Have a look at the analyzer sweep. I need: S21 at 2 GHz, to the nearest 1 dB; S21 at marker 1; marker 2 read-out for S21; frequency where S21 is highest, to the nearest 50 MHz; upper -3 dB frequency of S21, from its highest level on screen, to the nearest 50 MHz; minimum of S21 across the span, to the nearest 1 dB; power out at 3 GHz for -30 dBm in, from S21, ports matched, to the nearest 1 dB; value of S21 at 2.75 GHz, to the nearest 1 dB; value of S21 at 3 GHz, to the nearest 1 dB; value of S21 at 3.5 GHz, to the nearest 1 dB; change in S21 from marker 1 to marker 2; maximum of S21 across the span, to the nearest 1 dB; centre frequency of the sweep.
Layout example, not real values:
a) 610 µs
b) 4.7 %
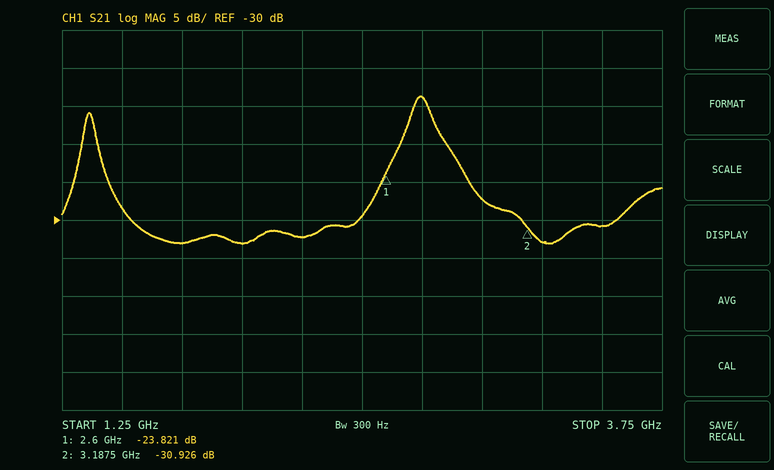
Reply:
a) -33 dB
b) -23.821 dB
c) -30.926 dB
d) 2.75 GHz
e) 2.80 GHz
f) -33 dB
g) -57 dBm
h) -14 dB
i) -27 dB
j) -31 dB
k) -7.105 dB
l) -14 dB
m) 2.5 GHz
